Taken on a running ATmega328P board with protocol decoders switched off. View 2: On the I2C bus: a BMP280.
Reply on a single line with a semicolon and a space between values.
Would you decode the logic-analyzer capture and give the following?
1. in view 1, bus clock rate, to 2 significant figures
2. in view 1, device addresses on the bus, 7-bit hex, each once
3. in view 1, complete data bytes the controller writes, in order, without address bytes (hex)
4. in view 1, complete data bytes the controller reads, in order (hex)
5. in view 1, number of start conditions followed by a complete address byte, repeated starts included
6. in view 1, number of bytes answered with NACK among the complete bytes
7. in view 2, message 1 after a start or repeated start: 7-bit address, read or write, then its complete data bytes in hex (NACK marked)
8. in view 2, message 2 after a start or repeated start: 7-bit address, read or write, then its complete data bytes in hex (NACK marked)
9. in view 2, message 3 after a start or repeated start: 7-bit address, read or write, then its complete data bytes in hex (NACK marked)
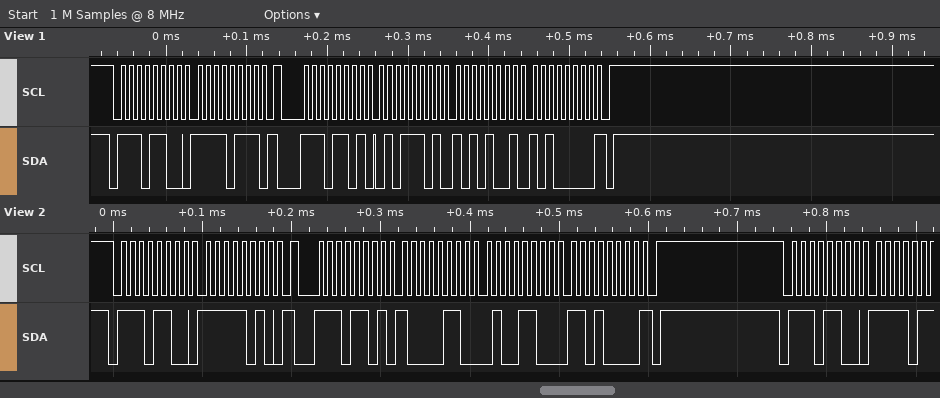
100 kHz; 0x76; F7; 5D A9 A0; 2; 1; 0x76 write: FA; 0x76 read: 86 4C D0 NACK; 0x76 write
